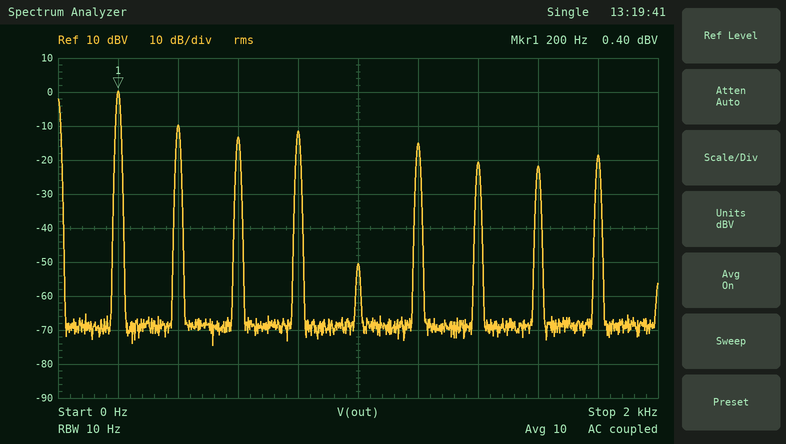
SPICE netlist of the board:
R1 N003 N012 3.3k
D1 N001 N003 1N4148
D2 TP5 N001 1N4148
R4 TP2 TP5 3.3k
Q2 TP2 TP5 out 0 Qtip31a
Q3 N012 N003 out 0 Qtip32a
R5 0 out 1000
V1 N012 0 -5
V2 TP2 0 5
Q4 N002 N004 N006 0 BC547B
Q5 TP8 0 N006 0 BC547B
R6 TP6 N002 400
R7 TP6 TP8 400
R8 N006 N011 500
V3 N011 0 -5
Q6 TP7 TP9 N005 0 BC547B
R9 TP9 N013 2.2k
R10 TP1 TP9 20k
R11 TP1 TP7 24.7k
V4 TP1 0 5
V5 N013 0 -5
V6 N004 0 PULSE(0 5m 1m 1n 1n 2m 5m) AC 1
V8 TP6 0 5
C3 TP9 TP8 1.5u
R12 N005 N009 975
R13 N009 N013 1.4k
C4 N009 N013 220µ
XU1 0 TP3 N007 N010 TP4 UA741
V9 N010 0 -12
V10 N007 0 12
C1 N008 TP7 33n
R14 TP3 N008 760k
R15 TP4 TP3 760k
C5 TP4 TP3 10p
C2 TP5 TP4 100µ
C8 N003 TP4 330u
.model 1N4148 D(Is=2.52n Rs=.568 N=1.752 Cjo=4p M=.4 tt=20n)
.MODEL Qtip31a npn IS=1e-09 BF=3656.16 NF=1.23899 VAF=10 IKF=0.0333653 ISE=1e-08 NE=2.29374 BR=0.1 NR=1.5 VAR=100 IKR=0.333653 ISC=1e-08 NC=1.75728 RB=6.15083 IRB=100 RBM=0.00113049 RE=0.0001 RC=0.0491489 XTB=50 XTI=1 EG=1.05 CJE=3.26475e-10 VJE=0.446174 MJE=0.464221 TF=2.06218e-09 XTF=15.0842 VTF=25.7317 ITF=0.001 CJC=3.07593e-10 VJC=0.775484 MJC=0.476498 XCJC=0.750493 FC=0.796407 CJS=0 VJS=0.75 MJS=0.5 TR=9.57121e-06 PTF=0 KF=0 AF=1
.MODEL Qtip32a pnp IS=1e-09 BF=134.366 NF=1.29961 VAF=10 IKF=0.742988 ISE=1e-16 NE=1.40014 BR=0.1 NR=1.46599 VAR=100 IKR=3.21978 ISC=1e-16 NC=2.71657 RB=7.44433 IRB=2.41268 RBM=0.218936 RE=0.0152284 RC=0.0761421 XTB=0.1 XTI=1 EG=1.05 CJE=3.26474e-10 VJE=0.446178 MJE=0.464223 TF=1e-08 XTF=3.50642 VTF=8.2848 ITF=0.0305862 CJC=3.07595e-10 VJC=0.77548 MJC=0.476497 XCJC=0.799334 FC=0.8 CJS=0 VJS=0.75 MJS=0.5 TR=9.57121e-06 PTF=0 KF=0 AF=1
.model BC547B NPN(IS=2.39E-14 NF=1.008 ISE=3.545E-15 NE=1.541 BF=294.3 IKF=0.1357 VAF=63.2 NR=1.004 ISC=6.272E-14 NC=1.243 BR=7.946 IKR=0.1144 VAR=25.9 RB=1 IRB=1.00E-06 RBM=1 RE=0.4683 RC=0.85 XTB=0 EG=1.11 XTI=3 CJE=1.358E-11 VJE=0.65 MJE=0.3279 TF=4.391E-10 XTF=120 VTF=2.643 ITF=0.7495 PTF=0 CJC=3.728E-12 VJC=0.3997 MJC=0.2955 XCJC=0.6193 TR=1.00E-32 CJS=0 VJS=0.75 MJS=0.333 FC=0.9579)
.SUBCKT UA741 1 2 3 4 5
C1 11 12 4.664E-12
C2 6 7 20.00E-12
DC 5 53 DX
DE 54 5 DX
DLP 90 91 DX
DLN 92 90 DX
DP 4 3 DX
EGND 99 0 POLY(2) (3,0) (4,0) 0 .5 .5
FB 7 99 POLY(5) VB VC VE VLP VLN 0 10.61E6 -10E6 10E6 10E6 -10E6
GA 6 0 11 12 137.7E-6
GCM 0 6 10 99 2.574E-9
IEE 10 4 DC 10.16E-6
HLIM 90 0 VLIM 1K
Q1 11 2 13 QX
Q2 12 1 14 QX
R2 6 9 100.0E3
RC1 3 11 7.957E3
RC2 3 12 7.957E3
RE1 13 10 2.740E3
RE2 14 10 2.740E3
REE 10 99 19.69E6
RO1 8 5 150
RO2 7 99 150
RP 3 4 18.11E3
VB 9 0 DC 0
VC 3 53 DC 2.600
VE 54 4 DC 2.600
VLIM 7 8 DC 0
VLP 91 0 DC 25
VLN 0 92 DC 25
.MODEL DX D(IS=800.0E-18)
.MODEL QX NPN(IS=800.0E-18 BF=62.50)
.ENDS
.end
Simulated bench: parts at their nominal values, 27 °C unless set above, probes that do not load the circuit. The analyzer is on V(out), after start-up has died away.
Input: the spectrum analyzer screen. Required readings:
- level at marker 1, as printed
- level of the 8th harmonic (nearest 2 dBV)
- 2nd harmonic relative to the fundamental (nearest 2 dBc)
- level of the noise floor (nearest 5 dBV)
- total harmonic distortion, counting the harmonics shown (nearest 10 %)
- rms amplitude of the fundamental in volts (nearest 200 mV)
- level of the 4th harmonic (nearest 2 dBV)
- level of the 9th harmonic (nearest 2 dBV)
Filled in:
0.40 dBV
-22 dBV
-10 dBc
-70 dBV
50 %
1.0 V
-12 dBV
-18 dBV
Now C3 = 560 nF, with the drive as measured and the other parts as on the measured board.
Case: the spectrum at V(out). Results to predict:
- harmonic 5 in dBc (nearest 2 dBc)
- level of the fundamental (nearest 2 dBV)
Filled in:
-42 dBc
0 dBV
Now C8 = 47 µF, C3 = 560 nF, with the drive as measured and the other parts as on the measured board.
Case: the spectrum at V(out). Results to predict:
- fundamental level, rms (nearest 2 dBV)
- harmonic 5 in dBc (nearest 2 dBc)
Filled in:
0 dBV
-42 dBc
